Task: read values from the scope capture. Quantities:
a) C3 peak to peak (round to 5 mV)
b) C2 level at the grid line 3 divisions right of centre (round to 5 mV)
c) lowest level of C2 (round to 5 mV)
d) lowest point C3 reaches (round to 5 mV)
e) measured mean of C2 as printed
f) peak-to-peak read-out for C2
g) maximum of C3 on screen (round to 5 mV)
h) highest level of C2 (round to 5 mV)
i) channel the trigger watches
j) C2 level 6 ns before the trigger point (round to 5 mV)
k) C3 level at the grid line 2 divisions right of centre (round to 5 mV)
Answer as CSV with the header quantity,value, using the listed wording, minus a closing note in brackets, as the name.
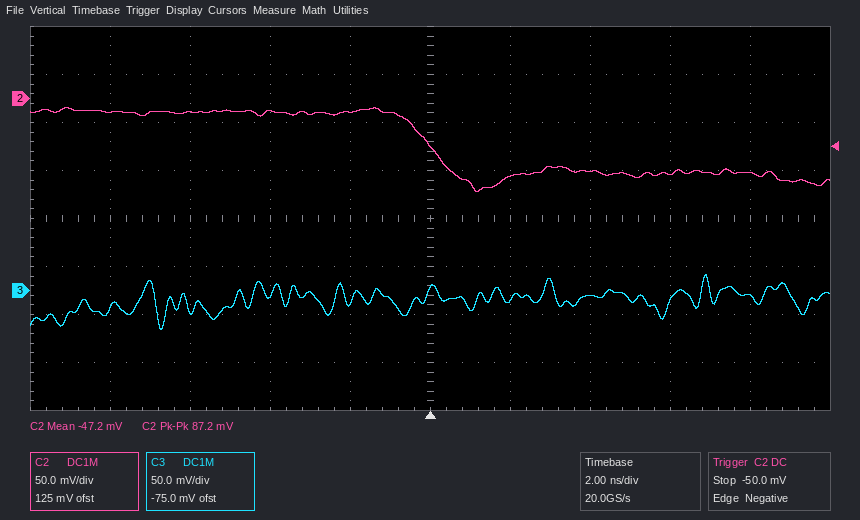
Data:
quantity,value
C3 peak to peak,55 mV
C2 level at the grid line 3 divisions right of centre,-80 mV
lowest level of C2,-95 mV
lowest point C3 reaches,-40 mV
measured mean of C2 as printed,-47.2 mV
peak-to-peak read-out for C2,87.2 mV
maximum of C3 on screen,15 mV
highest level of C2,-10 mV
channel the trigger watches,C2
C2 level 6 ns before the trigger point,-15 mV
C3 level at the grid line 2 divisions right of centre,-5 mV
